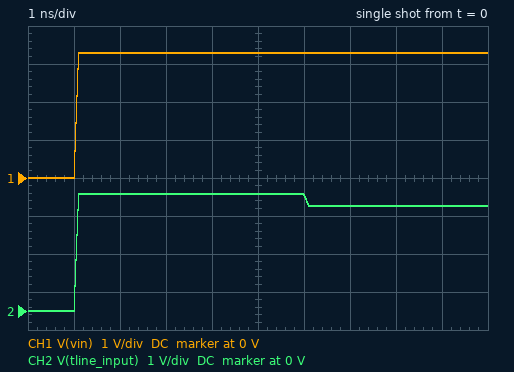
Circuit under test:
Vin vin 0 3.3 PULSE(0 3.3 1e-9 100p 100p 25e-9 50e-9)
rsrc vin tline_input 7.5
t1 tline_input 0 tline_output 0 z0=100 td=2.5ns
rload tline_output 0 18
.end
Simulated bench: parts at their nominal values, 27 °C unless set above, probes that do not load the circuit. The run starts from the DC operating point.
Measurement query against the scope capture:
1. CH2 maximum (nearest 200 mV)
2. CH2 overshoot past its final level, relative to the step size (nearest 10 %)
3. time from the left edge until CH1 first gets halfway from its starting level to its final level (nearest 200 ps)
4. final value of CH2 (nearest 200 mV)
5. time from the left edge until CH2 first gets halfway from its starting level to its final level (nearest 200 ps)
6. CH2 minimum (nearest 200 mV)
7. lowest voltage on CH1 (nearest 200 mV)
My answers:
3.0 V
10 %
1.0 ns
2.8 V
1.0 ns
0 V
0 V
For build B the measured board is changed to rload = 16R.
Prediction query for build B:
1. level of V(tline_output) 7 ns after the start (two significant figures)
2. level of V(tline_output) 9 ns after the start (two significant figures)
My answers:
850 mV
1.4 V
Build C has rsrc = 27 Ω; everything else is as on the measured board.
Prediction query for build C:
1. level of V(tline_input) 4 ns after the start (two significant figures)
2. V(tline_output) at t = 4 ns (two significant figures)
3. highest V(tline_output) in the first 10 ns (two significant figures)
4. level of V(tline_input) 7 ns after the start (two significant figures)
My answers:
2.6 V
790 mV
1.1 V
1.8 V
